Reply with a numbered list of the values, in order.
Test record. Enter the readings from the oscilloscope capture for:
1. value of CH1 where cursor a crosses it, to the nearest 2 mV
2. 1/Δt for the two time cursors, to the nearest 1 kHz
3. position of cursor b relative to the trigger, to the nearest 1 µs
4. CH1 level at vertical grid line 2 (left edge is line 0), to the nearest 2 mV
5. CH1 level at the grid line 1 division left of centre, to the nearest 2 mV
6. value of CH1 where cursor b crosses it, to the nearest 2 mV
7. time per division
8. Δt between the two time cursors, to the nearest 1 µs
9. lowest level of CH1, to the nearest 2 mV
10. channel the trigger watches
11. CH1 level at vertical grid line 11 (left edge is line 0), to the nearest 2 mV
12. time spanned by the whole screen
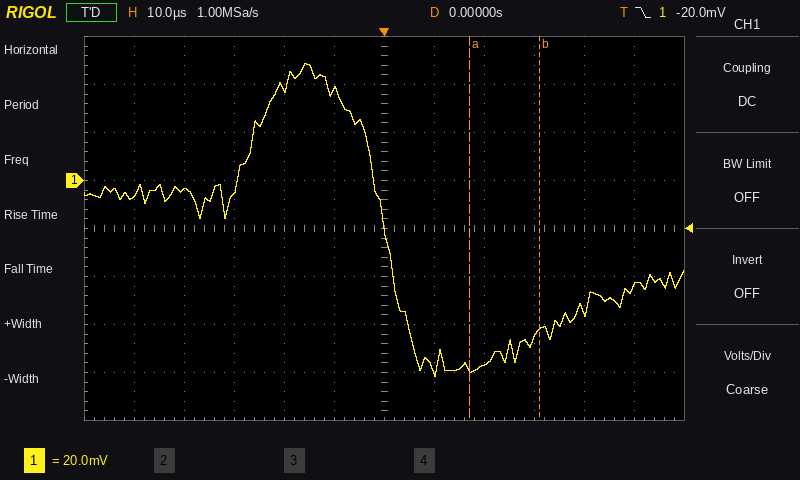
1. -78 mV
2. 71 kHz
3. +31 µs
4. -4 mV
5. 38 mV
6. -62 mV
7. 10 µs
8. 14 µs
9. -82 mV
10. CH1
11. -44 mV
12. 120 µs
